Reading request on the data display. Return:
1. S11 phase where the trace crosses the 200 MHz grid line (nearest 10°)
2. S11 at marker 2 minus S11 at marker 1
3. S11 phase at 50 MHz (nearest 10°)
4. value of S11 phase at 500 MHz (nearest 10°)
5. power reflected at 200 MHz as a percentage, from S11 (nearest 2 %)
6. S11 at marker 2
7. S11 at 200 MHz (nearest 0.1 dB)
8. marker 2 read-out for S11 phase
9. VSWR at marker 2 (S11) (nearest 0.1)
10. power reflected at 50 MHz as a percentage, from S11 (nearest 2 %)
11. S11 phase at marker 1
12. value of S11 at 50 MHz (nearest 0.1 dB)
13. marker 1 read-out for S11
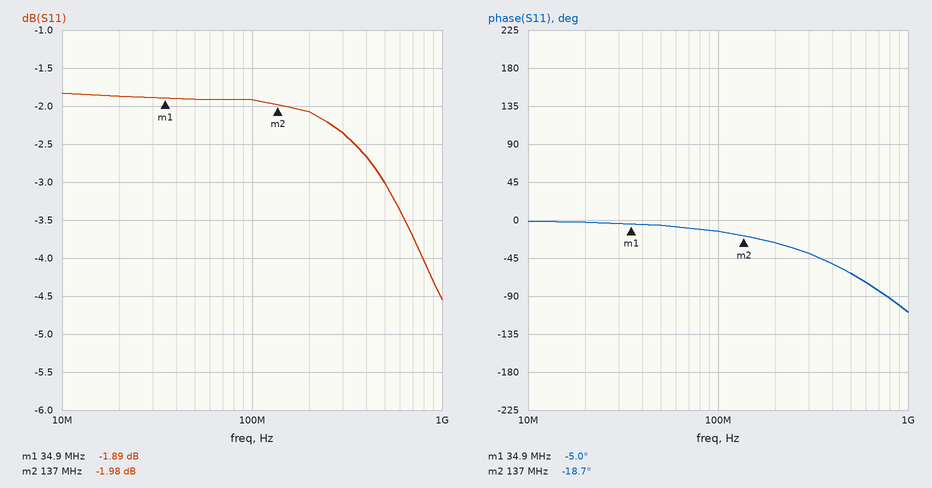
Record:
-30°
-0.09 dB
-10°
-60°
62 %
-1.98 dB
-2.1 dB
-18.7°
8.8
64 %
-5.0°
-1.9 dB
-1.89 dB
